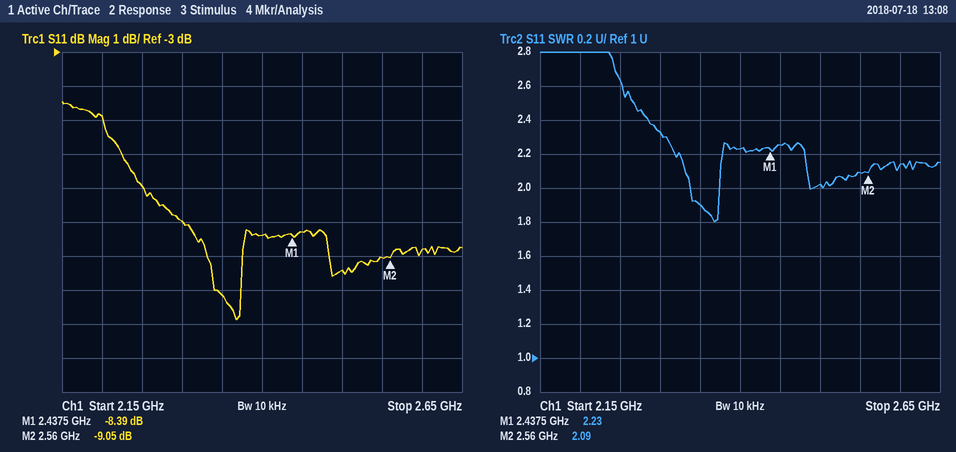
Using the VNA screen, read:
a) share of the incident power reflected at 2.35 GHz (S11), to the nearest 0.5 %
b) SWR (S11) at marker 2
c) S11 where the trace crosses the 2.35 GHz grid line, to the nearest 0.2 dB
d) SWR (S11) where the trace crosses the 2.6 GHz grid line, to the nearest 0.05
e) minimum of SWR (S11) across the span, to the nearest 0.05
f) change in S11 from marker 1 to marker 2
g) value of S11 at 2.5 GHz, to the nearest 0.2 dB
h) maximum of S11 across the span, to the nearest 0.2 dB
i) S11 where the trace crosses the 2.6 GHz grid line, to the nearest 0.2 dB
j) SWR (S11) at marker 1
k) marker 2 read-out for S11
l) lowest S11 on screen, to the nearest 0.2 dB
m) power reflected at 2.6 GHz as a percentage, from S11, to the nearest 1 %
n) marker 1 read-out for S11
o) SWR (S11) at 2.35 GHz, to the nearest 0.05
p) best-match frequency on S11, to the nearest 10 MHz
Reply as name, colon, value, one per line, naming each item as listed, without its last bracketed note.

share of the incident power reflected at 2.35 GHz (S11), to the nearest 0.5 %: 9.5 %
SWR (S11) at marker 2: 2.09
S11 where the trace crosses the 2.35 GHz grid line, to the nearest 0.2 dB: -10.2 dB
SWR (S11) where the trace crosses the 2.6 GHz grid line, to the nearest 0.05: 2.15
minimum of SWR (S11) across the span, to the nearest 0.05: 1.80
change in S11 from marker 1 to marker 2: -0.66 dB
value of S11 at 2.5 GHz, to the nearest 0.2 dB: -9.4 dB
maximum of S11 across the span, to the nearest 0.2 dB: -4.4 dB
S11 where the trace crosses the 2.6 GHz grid line, to the nearest 0.2 dB: -8.8 dB
SWR (S11) at marker 1: 2.23
marker 2 read-out for S11: -9.05 dB
lowest S11 on screen, to the nearest 0.2 dB: -10.8 dB
power reflected at 2.6 GHz as a percentage, from S11, to the nearest 1 %: 13 %
marker 1 read-out for S11: -8.39 dB
SWR (S11) at 2.35 GHz, to the nearest 0.05: 1.90
best-match frequency on S11, to the nearest 10 MHz: 2.37 GHz
